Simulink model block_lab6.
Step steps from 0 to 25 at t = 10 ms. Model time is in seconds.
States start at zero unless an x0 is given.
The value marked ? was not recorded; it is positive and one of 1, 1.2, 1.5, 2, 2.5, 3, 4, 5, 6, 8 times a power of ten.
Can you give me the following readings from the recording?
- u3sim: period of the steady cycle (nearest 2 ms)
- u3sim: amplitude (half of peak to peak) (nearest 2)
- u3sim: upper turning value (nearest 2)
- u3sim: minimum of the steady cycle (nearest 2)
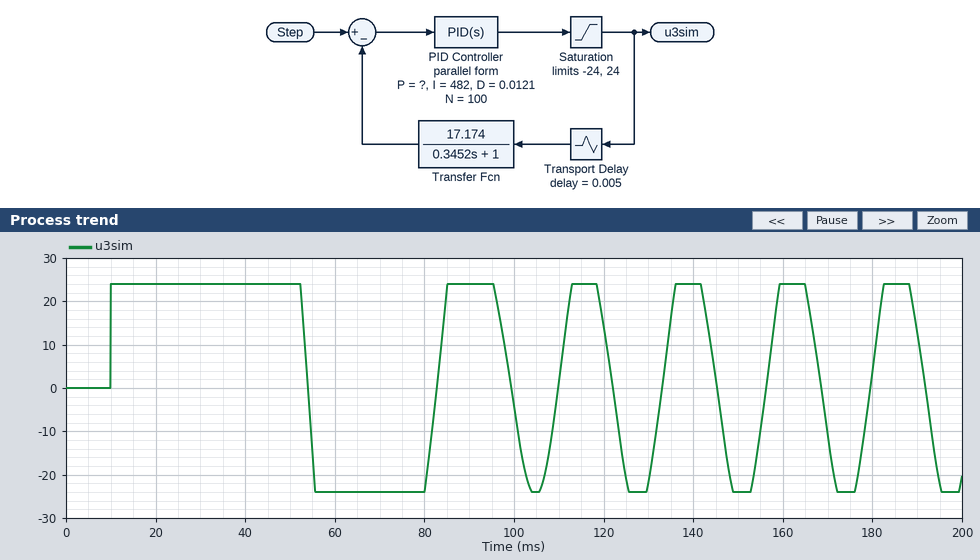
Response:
24 ms
24
24
-24
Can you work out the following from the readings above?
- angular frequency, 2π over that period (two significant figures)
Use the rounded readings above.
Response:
0.26 rad/ms
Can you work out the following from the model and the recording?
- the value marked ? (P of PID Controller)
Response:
5
